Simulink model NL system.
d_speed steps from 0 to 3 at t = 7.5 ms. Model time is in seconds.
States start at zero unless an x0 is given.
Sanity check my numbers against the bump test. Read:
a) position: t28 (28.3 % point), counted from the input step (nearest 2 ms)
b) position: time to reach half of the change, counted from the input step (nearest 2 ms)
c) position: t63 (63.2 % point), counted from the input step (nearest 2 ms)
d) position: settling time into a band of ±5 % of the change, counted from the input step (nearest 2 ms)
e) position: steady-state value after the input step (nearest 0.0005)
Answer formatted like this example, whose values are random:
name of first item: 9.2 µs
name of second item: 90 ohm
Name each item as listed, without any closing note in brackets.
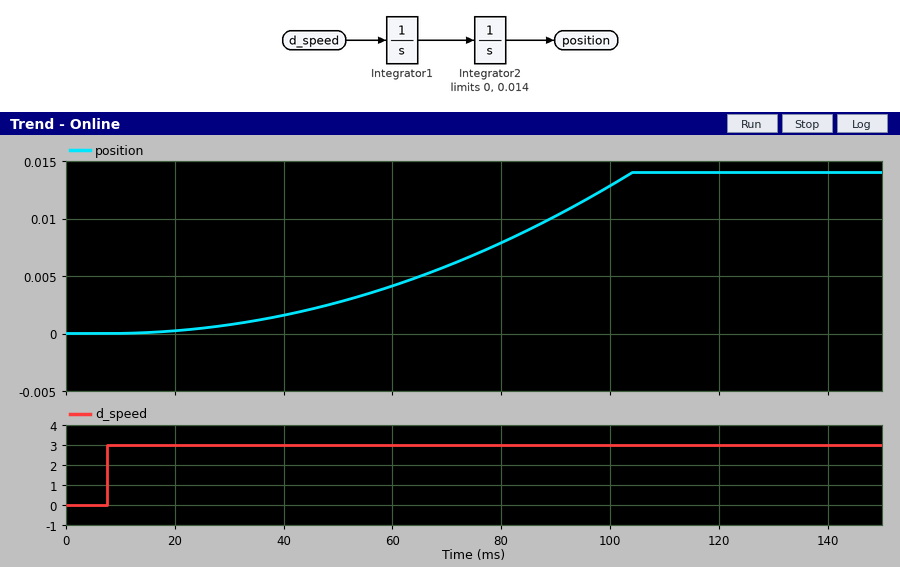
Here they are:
position: t28 (28.3 % point), counted from the input step: 52 ms
position: time to reach half of the change, counted from the input step: 68 ms
position: t63 (63.2 % point), counted from the input step: 76 ms
position: settling time into a band of ±5 % of the change, counted from the input step: 94 ms
position: steady-state value after the input step: 0.0140
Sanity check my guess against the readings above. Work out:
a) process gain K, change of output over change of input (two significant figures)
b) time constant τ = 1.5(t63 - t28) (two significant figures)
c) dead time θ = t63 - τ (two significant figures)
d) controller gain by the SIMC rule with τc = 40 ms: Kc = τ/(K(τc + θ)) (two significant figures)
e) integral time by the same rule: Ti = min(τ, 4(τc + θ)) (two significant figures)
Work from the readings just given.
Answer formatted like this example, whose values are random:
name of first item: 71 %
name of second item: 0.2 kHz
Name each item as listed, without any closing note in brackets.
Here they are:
process gain K, change of output over change of input: 0.0047
time constant τ = 1.5(t63 - t28): 36 ms
dead time θ = t63 - τ: 40 ms
controller gain by the SIMC rule with τc = 40 ms: Kc = τ/(K(τc + θ)): 96
integral time by the same rule: Ti = min(τ, 4(τc + θ)): 36 ms
